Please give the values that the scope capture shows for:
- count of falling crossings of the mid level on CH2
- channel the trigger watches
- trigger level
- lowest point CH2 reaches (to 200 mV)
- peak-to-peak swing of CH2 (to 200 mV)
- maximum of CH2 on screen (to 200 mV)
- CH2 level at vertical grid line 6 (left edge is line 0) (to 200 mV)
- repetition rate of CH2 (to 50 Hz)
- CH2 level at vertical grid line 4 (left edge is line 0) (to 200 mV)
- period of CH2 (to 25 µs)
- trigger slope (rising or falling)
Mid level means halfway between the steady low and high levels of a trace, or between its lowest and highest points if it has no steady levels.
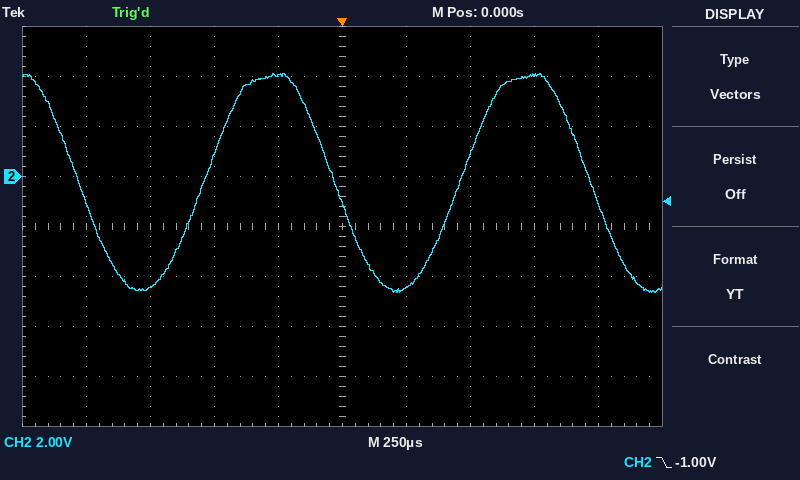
3
CH2
-1.00 V
-4.6 V
8.8 V
4.2 V
-4.4 V
1.00 kHz
4.0 V
1.000 ms
falling
